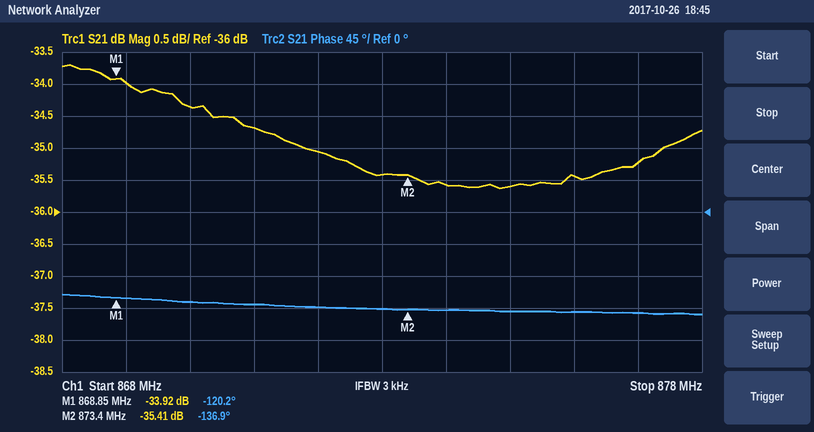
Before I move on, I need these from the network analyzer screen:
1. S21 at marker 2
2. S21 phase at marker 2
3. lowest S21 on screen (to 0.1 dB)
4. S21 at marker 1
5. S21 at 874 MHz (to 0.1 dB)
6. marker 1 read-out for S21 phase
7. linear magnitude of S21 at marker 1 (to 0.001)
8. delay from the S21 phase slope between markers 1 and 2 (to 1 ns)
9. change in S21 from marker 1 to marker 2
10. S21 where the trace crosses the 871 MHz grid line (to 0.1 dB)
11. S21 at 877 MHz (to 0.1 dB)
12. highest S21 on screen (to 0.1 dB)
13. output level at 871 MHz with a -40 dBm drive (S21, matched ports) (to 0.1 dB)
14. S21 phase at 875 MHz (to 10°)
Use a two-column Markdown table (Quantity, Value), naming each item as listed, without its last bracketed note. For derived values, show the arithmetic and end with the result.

| Quantity | Value |
|---|---|
| S21 at marker 2 | -35.41 dB |
| S21 phase at marker 2 | -136.9° |
| lowest S21 on screen | -35.6 dB |
| S21 at marker 1 | -33.92 dB |
| S21 at 874 MHz | -35.6 dB |
| marker 1 read-out for S21 phase | -120.2° |
| linear magnitude of S21 at marker 1 | 10^(-33.92/20) ≈ 0.020 |
| delay from the S21 phase slope between markers 1 and 2 | −(-136.9° − (-120.2°))/(360° × 4.55 MHz) ≈ 10 ns |
| change in S21 from marker 1 to marker 2 | -35.41 − (-33.92) = -1.49 dB |
| S21 where the trace crosses the 871 MHz grid line | -34.7 dB |
| S21 at 877 MHz | -35.2 dB |
| highest S21 on screen | -33.7 dB |
| output level at 871 MHz with a -40 dBm drive (S21, matched ports) | -40 dBm + (-34.7 dB) = -74.7 dBm |
| S21 phase at 875 MHz | -140° |
